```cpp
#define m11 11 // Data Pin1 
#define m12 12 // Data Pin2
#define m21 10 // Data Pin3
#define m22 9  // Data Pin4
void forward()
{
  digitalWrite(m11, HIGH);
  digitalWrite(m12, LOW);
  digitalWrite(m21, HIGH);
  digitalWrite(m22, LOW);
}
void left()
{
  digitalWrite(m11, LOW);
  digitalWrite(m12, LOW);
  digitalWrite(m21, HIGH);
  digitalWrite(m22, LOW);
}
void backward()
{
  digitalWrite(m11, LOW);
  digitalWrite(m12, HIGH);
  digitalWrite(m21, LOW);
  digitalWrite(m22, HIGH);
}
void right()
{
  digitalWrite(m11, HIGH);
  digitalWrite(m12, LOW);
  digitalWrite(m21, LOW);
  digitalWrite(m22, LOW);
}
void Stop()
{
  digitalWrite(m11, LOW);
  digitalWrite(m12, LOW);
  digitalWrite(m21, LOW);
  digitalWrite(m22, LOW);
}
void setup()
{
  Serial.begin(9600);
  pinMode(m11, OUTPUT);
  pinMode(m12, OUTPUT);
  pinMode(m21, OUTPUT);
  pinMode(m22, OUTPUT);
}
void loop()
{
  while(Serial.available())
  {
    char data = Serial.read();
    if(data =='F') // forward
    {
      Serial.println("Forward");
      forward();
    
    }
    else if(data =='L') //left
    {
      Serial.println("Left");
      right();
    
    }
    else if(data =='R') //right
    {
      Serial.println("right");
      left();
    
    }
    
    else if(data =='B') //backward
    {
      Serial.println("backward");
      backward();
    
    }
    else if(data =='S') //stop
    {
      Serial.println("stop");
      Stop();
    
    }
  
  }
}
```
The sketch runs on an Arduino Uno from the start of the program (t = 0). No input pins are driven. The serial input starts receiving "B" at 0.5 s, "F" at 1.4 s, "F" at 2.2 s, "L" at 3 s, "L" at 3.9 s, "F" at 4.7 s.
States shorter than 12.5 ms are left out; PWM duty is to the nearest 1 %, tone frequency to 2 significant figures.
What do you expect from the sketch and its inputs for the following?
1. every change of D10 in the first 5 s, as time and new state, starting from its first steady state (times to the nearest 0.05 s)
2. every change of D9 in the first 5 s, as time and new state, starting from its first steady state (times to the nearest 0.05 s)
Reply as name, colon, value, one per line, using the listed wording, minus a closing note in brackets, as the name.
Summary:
every change of D10 in the first 5 s, as time and new state, starting from its first steady state: 0 s low; 1.4 s high; 3 s low; 4.7 s high
every change of D9 in the first 5 s, as time and new state, starting from its first steady state: 0 s low; 0.5 s high; 1.4 s low
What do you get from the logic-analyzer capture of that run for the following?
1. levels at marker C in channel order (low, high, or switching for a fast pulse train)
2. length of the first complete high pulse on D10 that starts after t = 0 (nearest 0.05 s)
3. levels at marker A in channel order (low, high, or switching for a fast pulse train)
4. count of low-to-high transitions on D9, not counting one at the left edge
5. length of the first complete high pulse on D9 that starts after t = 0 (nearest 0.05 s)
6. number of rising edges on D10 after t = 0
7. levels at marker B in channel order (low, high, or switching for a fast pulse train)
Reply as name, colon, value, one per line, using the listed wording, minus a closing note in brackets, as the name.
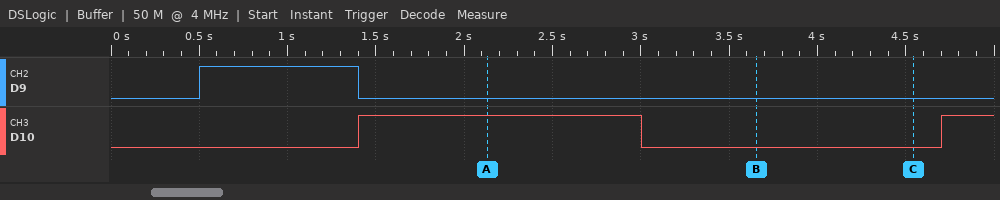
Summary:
levels at marker C in channel order: D9 low, D10 low
length of the first complete high pulse on D10 that starts after t = 0: 1.60 s
levels at marker A in channel order: D9 low, D10 high
count of low-to-high transitions on D9, not counting one at the left edge: 1
length of the first complete high pulse on D9 that starts after t = 0: 0.90 s
number of rising edges on D10 after t = 0: 2
levels at marker B in channel order: D9 low, D10 low
